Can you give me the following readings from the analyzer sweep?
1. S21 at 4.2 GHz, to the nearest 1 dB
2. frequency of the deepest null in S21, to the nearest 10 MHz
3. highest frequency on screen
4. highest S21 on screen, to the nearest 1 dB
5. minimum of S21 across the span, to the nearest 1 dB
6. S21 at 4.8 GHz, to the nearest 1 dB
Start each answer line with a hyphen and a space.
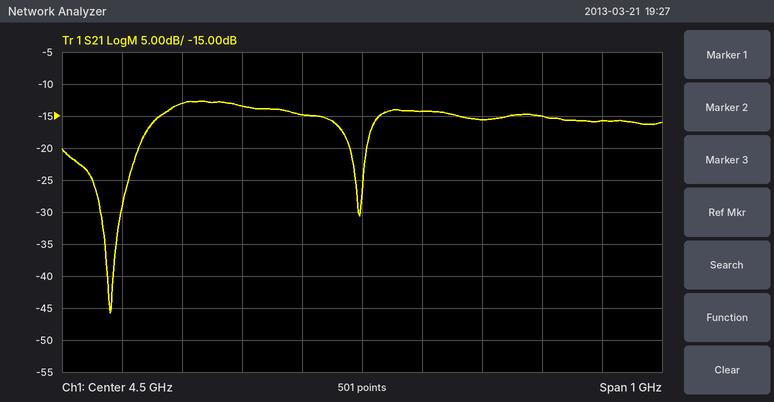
- -13 dB
- 4.08 GHz
- 5 GHz
- -13 dB
- -46 dB
- -15 dB
